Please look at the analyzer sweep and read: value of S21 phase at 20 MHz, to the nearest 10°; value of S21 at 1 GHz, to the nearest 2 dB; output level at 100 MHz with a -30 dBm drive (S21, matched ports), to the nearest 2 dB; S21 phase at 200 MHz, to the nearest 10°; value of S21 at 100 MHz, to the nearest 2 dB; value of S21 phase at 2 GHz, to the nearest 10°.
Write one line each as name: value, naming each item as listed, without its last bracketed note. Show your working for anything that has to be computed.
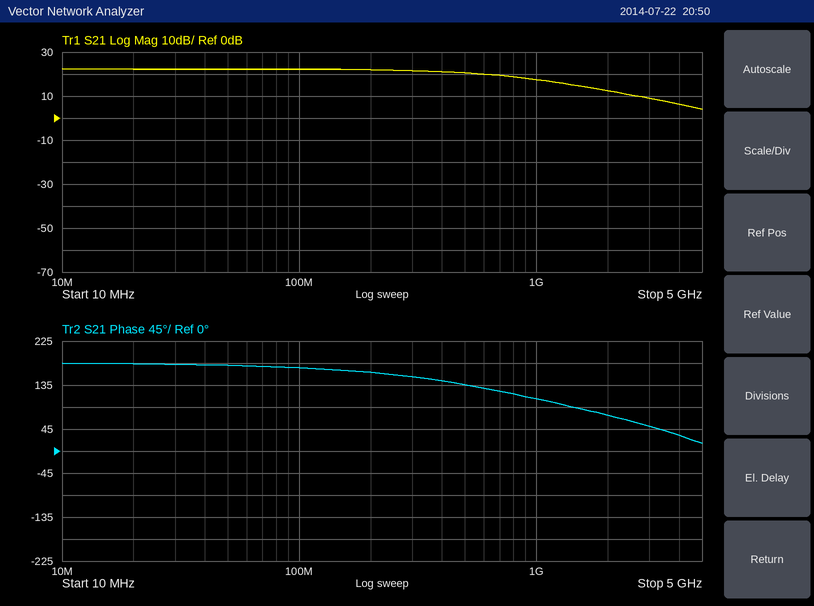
value of S21 phase at 20 MHz, to the nearest 10°: 180°
value of S21 at 1 GHz, to the nearest 2 dB: 18 dB
output level at 100 MHz with a -30 dBm drive (S21, matched ports), to the nearest 2 dB: -30 dBm + (22 dB) = -8 dBm
S21 phase at 200 MHz, to the nearest 10°: 160°
value of S21 at 100 MHz, to the nearest 2 dB: 22 dB
value of S21 phase at 2 GHz, to the nearest 10°: 70°
